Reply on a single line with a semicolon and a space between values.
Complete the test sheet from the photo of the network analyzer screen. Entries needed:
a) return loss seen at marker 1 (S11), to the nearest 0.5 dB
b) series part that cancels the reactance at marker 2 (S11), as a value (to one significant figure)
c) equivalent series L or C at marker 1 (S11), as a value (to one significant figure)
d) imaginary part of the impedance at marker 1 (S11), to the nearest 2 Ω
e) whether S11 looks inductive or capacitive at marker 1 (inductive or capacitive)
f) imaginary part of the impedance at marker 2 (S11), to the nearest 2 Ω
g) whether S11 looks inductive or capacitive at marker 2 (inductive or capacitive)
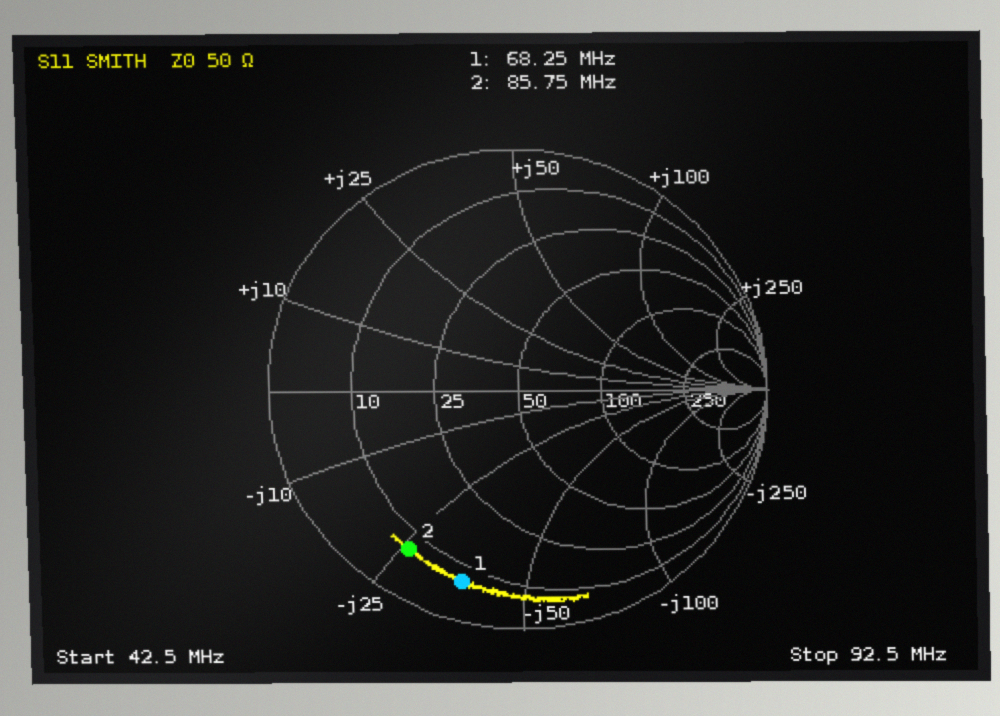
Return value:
1.5 dB; 50 nH; 60 pF; -36 Ω; capacitive; -26 Ω; capacitive
